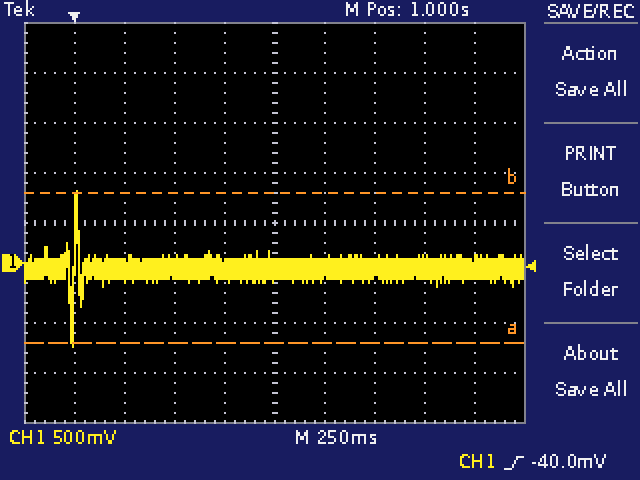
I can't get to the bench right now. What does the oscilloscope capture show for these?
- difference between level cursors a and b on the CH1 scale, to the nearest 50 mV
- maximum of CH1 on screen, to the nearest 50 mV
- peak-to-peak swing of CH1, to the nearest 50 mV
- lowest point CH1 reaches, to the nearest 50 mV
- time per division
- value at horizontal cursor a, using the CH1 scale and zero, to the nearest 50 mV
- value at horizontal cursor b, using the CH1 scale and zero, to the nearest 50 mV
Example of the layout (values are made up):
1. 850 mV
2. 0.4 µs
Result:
1. 1.50 V
2. 700 mV
3. 1.55 V
4. -850 mV
5. 250 ms
6. -800 mV
7. 700 mV
